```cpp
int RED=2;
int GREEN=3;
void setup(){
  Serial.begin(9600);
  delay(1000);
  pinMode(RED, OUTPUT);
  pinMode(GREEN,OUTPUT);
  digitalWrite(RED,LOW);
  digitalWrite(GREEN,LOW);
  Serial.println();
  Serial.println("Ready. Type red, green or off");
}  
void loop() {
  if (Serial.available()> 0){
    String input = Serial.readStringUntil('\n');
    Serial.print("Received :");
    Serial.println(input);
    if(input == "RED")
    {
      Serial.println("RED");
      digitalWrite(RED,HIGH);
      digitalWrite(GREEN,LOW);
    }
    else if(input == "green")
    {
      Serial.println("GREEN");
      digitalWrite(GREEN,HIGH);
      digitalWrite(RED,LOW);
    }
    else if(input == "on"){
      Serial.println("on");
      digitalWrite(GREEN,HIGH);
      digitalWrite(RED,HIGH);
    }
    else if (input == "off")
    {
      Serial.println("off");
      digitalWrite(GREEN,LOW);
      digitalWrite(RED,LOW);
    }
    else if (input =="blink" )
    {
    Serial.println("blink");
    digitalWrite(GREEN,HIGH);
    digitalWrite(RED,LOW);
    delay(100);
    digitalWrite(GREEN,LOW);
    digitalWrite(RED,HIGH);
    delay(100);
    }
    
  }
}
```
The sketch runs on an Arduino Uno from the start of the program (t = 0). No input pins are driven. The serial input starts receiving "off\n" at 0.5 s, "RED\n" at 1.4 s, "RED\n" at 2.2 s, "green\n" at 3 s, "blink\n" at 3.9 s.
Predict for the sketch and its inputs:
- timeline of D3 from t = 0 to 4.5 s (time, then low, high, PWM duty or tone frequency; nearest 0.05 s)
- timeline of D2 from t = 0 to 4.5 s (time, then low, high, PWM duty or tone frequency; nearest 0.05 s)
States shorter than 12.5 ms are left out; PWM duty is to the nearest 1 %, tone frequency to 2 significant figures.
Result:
1 s low; 3 s high; 4 s low
1 s low; 1.4 s high; 3 s low; 4 s high
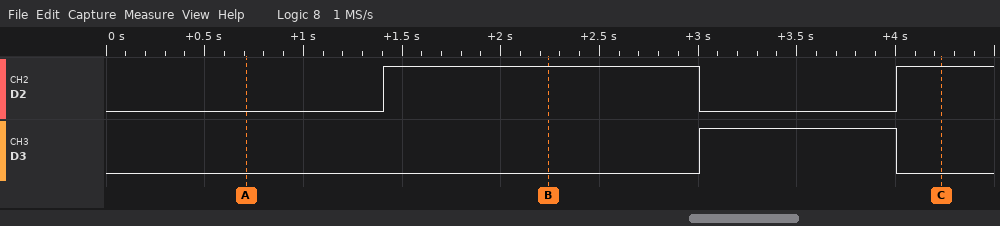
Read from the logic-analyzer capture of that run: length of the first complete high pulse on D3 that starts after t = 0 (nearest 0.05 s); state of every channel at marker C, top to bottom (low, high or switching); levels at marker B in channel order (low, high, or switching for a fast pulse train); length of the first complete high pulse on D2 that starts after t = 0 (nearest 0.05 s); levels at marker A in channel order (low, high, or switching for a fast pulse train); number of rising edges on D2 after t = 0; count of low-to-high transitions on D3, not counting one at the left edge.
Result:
1.00 s
D2 high, D3 low
D2 high, D3 low
1.60 s
D2 low, D3 low
2
1
